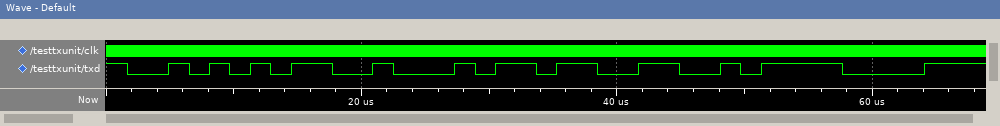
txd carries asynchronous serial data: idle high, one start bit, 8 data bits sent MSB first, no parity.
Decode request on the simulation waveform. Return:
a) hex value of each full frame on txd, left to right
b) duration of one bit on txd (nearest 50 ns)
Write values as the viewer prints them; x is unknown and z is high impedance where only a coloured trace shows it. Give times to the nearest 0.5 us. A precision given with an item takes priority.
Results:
55, 45, CC, F0
1600 ns
